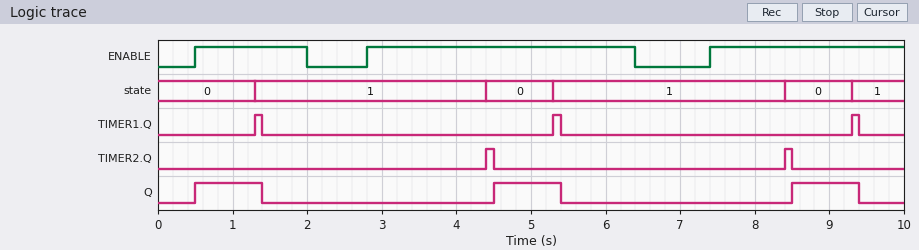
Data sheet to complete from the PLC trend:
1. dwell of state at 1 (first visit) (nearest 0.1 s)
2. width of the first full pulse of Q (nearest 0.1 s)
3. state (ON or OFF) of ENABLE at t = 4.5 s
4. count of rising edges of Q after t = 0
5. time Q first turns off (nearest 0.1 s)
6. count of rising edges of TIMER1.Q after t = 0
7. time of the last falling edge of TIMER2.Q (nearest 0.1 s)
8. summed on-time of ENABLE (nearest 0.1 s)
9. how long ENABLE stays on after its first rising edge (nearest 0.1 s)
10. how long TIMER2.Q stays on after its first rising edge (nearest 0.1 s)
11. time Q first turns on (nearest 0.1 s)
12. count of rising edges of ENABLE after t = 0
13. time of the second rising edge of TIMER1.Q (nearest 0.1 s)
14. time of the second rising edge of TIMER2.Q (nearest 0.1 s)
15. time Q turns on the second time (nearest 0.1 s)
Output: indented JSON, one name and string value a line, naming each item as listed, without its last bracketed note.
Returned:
{
  "dwell of state at 1 (first visit)": "3.1 s",
  "width of the first full pulse of Q": "0.9 s",
  "state (ON or OFF) of ENABLE at t = 4.5 s": "ON",
  "count of rising edges of Q after t = 0": "3",
  "time Q first turns off": "1.4 s",
  "count of rising edges of TIMER1.Q after t = 0": "3",
  "time of the last falling edge of TIMER2.Q": "8.5 s",
  "summed on-time of ENABLE": "7.7 s",
  "how long ENABLE stays on after its first rising edge": "1.5 s",
  "how long TIMER2.Q stays on after its first rising edge": "0.1 s",
  "time Q first turns on": "0.5 s",
  "count of rising edges of ENABLE after t = 0": "3",
  "time of the second rising edge of TIMER1.Q": "5.3 s",
  "time of the second rising edge of TIMER2.Q": "8.4 s",
  "time Q turns on the second time": "4.5 s"
}
